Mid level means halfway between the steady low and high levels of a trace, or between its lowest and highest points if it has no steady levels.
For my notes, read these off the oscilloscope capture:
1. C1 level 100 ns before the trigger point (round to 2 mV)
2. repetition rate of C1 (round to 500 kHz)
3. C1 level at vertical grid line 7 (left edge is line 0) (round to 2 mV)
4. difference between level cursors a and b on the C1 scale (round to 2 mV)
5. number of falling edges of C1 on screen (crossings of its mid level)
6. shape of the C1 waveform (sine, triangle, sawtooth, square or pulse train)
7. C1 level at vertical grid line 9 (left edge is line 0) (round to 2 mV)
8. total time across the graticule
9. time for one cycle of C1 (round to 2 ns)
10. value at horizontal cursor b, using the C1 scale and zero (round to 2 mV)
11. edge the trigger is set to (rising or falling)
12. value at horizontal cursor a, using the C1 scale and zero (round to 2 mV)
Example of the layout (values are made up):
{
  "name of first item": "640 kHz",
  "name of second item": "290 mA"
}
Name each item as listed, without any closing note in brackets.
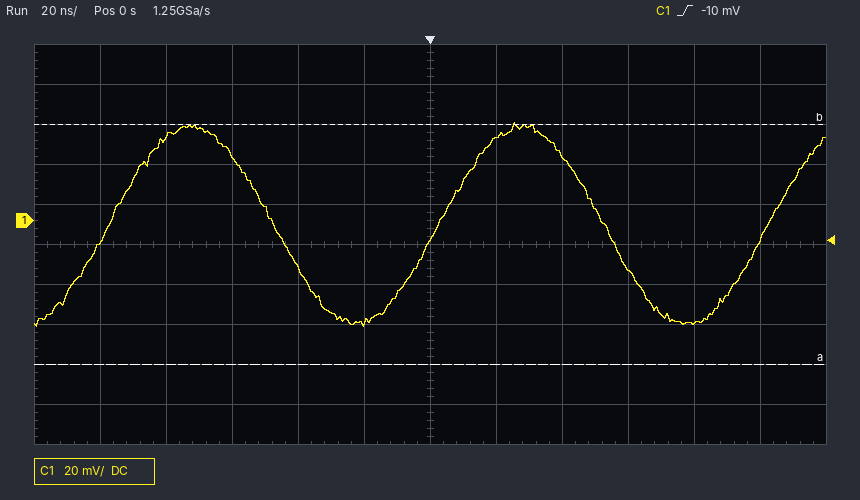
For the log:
{
  "C1 level 100 ns before the trigger point": "-10 mV",
  "repetition rate of C1": "10.0 MHz",
  "C1 level at vertical grid line 7 (left edge is line 0)": "42 mV",
  "difference between level cursors a and b on the C1 scale": "120 mV",
  "number of falling edges of C1 on screen": "2",
  "shape of the C1 waveform": "sine",
  "C1 level at vertical grid line 9 (left edge is line 0)": "-24 mV",
  "total time across the graticule": "240 ns",
  "time for one cycle of C1": "100 ns",
  "value at horizontal cursor b, using the C1 scale and zero": "48 mV",
  "edge the trigger is set to": "rising",
  "value at horizontal cursor a, using the C1 scale and zero": "-72 mV"
}
